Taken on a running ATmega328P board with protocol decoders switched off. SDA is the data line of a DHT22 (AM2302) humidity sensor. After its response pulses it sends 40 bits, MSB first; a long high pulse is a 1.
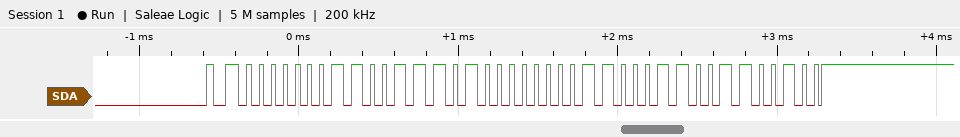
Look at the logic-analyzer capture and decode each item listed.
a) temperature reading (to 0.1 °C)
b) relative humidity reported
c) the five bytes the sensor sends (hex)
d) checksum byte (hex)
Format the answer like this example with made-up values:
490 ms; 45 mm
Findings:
19.8 °C; 41.3 %; 01 9D 00 C6 64; 0x64
